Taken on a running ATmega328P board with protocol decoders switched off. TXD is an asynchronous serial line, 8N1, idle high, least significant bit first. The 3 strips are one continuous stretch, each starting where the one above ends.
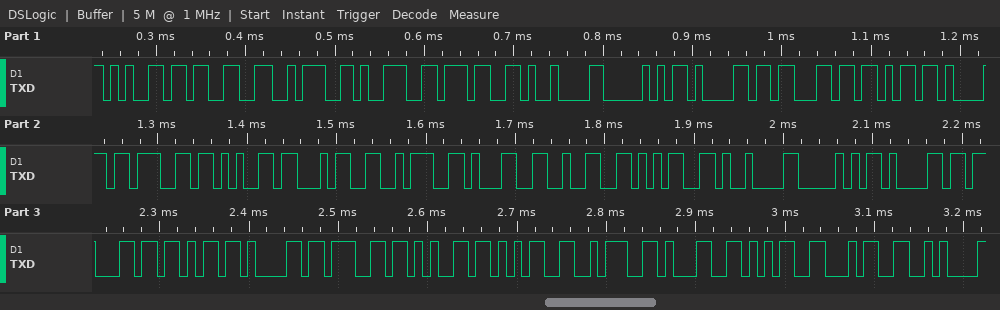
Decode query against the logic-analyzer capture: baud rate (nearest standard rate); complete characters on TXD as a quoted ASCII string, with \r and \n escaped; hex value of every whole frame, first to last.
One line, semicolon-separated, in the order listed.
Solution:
115200 baud; "e3:97\tPackage4:125\tPackage5:154\n"; 65 33 3A 39 37 09 50 61 63 6B 61 67 65 34 3A 31 32 35 09 50 61 63 6B 61 67 65 35 3A 31 35 34 0A
